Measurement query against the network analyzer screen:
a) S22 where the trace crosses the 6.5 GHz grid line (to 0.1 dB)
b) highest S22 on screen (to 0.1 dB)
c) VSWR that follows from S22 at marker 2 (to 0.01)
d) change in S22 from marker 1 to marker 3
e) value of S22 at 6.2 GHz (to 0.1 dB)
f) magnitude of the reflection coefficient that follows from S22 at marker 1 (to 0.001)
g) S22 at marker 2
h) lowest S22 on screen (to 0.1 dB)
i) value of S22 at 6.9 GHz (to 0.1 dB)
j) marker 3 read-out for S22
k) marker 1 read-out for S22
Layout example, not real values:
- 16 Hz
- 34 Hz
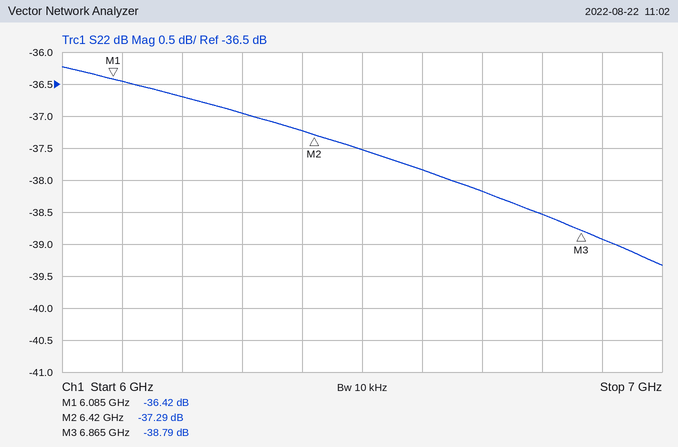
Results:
- -37.5 dB
- -36.2 dB
- 1.03
- -2.37 dB
- -36.7 dB
- 0.015
- -37.29 dB
- -39.3 dB
- -38.9 dB
- -38.79 dB
- -36.42 dB
